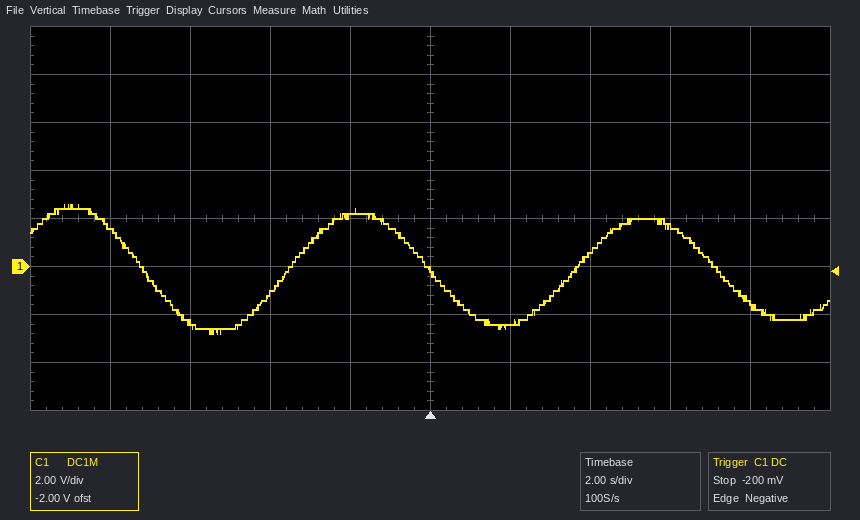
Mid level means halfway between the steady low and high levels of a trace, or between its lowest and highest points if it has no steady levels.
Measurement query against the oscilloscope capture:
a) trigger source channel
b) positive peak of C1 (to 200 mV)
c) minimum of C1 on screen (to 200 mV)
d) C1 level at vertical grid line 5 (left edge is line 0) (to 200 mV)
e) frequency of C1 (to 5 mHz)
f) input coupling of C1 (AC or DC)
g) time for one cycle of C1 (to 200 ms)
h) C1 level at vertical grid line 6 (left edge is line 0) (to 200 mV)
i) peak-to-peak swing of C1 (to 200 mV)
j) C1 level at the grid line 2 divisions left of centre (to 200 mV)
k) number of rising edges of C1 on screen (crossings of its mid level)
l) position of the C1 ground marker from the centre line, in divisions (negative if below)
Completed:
C1
2.6 V
-2.8 V
-200 mV
140 mHz
DC
7.2 s
-2.4 V
5.4 V
-1.2 V
2
-1.0 div
